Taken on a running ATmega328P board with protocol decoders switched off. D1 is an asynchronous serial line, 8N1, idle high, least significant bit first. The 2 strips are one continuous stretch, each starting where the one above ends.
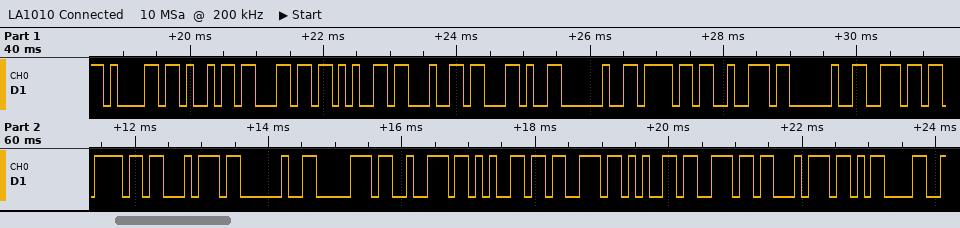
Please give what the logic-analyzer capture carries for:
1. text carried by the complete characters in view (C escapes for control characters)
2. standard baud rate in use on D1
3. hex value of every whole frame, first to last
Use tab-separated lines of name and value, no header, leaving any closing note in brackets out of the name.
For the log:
text carried by the complete characters in view	"ailed, or not present\r"
standard baud rate in use on D1	9600 baud
hex value of every whole frame, first to last	61 69 6C 65 64 2C 20 6F 72 20 6E 6F 74 20 70 72 65 73 65 6E 74 0D
